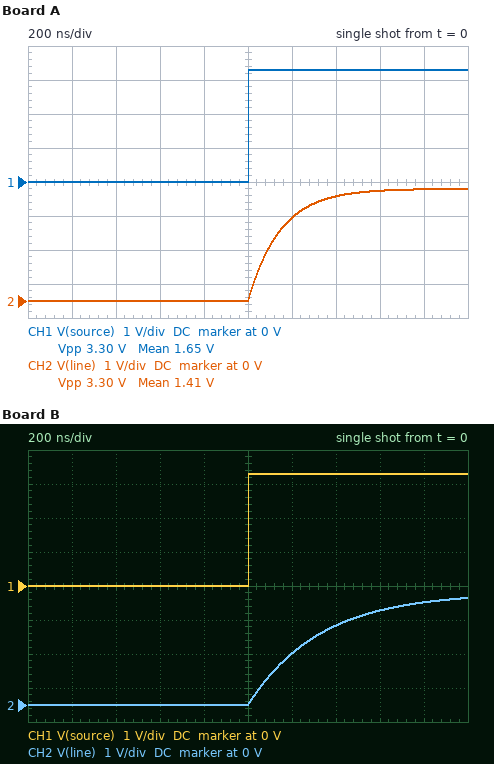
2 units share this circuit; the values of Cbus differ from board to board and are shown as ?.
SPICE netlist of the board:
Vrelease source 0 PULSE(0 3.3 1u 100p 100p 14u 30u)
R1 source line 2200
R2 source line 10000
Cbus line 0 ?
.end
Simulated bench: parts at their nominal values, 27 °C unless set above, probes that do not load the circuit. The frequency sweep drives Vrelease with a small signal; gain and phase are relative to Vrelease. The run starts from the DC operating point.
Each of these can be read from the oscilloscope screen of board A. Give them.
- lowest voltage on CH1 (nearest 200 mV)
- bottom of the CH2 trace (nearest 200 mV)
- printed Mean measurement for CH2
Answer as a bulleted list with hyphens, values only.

- 0 V
- 0 V
- 1.41 V
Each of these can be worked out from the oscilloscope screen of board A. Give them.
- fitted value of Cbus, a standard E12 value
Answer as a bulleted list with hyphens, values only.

- 82 pF
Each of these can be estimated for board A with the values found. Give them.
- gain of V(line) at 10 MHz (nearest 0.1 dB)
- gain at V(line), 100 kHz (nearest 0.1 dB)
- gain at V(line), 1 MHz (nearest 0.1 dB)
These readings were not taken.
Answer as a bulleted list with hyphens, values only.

- -19.4 dB
- 0 dB
- -2.7 dB
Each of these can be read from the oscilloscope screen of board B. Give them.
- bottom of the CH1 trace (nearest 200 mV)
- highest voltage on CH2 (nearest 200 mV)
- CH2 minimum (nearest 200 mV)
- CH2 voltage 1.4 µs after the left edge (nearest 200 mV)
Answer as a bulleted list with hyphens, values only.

- 0 V
- 3.2 V
- 0 V
- 2.4 V
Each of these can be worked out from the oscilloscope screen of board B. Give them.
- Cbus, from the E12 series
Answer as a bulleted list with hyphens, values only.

- 180 pF
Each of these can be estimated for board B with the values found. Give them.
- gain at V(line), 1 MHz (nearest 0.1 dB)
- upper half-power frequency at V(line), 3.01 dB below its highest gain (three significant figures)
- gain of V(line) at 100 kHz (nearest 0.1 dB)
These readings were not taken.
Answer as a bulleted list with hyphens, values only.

- -7.1 dB
- 490 kHz
- -0.2 dB
